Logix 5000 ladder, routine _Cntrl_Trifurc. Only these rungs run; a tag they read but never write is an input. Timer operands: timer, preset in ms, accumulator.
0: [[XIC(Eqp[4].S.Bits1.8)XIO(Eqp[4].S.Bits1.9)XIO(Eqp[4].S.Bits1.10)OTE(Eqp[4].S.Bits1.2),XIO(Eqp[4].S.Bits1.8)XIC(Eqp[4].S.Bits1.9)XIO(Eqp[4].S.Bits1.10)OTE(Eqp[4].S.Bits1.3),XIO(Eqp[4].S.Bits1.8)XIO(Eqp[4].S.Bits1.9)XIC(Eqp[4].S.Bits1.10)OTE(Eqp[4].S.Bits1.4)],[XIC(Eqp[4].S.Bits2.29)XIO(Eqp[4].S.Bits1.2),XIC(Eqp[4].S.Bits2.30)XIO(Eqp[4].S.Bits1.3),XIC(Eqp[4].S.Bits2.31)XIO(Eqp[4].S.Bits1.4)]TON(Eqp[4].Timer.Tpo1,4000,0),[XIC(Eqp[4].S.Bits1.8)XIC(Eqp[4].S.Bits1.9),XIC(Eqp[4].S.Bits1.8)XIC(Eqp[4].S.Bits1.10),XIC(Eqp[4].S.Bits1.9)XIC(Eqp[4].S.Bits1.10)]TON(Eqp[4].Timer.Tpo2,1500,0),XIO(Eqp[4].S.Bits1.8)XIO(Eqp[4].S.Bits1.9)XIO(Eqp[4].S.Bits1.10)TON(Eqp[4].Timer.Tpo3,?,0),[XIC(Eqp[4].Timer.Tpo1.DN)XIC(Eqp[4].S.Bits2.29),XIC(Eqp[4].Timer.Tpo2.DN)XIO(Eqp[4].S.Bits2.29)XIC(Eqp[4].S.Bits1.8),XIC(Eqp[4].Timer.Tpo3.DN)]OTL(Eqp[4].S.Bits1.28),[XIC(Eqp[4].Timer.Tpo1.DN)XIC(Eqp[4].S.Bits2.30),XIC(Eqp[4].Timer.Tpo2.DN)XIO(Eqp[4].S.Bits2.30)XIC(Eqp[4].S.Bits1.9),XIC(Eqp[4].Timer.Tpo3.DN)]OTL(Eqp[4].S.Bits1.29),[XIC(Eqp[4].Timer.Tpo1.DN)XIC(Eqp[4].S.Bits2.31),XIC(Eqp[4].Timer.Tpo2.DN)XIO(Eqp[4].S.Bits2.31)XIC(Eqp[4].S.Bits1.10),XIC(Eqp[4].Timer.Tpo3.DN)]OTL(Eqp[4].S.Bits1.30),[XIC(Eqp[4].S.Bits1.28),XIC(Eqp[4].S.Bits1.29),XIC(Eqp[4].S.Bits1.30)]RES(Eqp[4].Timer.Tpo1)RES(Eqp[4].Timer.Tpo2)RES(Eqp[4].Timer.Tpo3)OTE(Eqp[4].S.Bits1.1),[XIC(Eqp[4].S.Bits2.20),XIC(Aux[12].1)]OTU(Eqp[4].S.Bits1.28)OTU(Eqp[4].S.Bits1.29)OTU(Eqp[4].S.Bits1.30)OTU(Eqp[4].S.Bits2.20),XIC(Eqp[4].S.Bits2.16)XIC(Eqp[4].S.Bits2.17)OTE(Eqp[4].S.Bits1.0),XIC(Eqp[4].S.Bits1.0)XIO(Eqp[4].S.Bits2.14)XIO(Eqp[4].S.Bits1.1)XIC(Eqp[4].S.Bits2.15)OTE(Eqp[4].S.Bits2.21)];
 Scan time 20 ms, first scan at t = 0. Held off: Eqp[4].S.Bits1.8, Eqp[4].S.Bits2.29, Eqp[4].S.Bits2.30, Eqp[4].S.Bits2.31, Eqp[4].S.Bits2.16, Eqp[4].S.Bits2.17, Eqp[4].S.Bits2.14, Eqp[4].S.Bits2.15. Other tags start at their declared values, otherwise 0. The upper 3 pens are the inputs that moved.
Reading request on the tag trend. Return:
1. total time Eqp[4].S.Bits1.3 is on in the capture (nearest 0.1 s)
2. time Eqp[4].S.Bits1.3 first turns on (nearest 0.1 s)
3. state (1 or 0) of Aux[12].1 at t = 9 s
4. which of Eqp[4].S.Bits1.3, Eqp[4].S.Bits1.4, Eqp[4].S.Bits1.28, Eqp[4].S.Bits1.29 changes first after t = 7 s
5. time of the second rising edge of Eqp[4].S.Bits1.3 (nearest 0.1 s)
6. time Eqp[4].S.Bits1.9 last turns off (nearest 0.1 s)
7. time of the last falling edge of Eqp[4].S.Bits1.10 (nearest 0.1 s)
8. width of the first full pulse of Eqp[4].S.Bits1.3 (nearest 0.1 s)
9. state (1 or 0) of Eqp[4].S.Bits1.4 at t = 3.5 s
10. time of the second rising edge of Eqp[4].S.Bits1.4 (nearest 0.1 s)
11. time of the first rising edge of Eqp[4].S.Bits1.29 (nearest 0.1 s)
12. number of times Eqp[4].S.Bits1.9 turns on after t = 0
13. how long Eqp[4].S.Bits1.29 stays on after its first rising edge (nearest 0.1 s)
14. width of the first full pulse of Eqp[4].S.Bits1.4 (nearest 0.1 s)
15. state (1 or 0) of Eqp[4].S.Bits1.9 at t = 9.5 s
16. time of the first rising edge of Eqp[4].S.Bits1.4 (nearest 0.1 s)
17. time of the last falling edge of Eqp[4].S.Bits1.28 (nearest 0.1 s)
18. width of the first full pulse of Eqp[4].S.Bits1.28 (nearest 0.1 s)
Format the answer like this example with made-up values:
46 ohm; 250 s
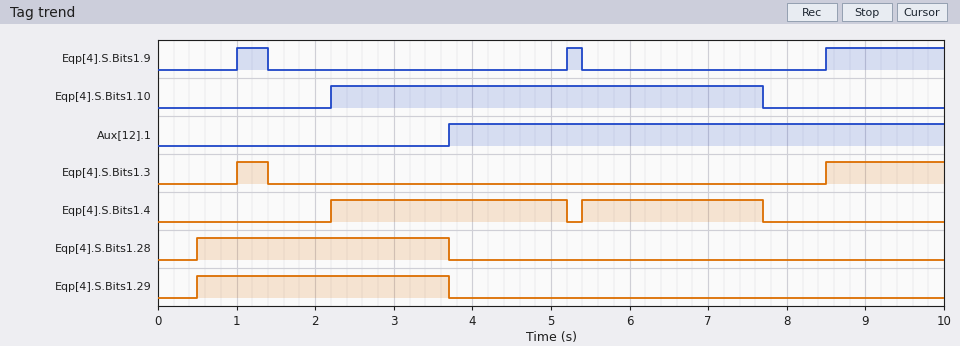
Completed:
1.9 s; 1.0 s; 1; Eqp[4].S.Bits1.4; 8.5 s; 5.4 s; 7.7 s; 0.4 s; 1; 5.4 s; 0.5 s; 3; 3.2 s; 3.0 s; 1; 2.2 s; 3.7 s; 3.2 s
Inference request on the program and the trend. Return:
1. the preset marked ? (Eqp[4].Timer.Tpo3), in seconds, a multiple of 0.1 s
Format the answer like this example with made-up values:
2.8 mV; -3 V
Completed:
0.5 s
